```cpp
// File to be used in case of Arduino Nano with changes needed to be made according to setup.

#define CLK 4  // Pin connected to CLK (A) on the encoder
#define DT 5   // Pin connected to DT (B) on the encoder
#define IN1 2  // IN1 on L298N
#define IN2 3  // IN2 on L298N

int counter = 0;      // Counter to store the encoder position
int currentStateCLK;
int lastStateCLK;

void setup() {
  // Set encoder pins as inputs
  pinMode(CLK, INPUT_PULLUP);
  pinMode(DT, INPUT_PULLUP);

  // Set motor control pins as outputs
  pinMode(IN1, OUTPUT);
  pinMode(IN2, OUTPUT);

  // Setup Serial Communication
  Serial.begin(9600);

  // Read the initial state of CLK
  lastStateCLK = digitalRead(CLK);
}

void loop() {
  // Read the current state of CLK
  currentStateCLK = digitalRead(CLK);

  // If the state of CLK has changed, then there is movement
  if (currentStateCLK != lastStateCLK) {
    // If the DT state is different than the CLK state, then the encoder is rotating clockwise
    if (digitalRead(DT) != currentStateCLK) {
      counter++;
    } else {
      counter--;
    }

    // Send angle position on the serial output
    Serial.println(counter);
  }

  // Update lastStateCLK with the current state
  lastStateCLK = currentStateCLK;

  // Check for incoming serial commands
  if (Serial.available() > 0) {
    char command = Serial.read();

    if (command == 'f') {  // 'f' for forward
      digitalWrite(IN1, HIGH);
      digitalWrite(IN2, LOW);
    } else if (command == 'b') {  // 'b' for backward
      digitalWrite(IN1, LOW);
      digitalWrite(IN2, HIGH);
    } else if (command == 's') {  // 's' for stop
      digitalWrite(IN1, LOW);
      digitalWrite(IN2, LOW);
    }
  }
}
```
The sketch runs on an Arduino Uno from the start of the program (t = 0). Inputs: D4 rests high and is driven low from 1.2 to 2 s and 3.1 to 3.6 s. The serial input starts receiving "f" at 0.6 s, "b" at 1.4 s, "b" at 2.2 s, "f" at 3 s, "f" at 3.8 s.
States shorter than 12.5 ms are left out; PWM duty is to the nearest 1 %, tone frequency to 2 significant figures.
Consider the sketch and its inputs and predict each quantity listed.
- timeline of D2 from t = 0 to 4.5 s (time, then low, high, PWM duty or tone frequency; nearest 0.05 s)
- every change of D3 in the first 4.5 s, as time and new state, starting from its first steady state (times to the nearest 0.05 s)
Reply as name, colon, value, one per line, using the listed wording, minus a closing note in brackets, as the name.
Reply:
timeline of D2 from t = 0 to 4.5 s: 0 s low; 0.6 s high; 1.4 s low; 3 s high
every change of D3 in the first 4.5 s, as time and new state, starting from its first steady state: 0 s low; 1.4 s high; 3 s low
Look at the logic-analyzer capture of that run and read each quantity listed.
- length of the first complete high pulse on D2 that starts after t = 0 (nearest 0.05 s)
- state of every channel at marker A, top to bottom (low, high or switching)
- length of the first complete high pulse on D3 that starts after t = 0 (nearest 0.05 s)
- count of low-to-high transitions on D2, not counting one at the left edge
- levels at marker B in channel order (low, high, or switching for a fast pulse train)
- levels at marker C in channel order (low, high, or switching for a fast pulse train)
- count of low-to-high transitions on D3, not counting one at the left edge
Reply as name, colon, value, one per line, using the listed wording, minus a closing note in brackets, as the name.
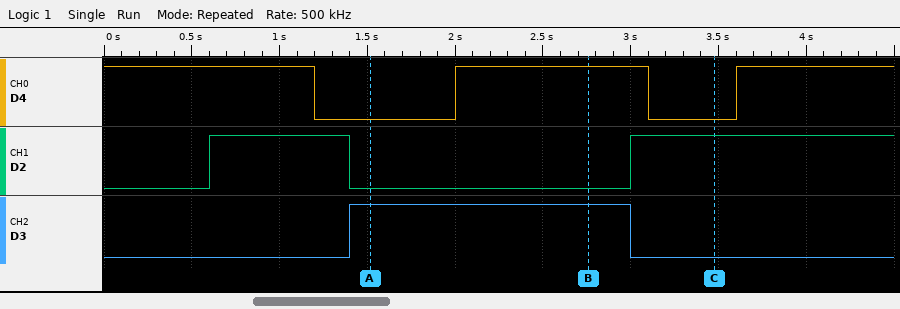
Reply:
length of the first complete high pulse on D2 that starts after t = 0: 0.80 s
state of every channel at marker A, top to bottom: D4 low, D2 low, D3 high
length of the first complete high pulse on D3 that starts after t = 0: 1.60 s
count of low-to-high transitions on D2, not counting one at the left edge: 2
levels at marker B in channel order: D4 high, D2 low, D3 high
levels at marker C in channel order: D4 low, D2 high, D3 low
count of low-to-high transitions on D3, not counting one at the left edge: 1
